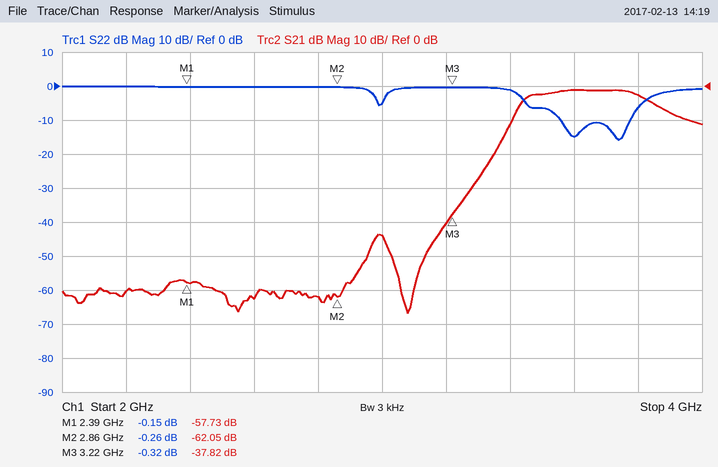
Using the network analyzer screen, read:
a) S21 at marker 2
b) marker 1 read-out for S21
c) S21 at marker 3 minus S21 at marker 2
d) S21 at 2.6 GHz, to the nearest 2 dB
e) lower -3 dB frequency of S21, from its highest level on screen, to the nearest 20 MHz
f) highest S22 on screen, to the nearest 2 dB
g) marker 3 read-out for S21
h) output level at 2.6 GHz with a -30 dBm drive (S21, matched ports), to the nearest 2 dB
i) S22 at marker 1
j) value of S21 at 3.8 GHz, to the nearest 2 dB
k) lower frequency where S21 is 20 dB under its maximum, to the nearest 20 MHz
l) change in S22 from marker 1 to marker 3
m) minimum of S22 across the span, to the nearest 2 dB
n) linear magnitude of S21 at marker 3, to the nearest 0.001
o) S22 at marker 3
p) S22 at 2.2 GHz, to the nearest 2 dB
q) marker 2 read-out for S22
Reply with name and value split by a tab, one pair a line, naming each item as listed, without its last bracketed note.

S21 at marker 2	-62.05 dB
marker 1 read-out for S21	-57.73 dB
S21 at marker 3 minus S21 at marker 2	24.23 dB
S21 at 2.6 GHz, to the nearest 2 dB	-62 dB
lower -3 dB frequency of S21, from its highest level on screen, to the nearest 20 MHz	3.44 GHz
highest S22 on screen, to the nearest 2 dB	0 dB
marker 3 read-out for S21	-37.82 dB
output level at 2.6 GHz with a -30 dBm drive (S21, matched ports), to the nearest 2 dB	-92 dBm
S22 at marker 1	-0.15 dB
value of S21 at 3.8 GHz, to the nearest 2 dB	-2 dB
lower frequency where S21 is 20 dB under its maximum, to the nearest 20 MHz	3.34 GHz
change in S22 from marker 1 to marker 3	-0.17 dB
minimum of S22 across the span, to the nearest 2 dB	-16 dB
linear magnitude of S21 at marker 3, to the nearest 0.001	0.013
S22 at marker 3	-0.32 dB
S22 at 2.2 GHz, to the nearest 2 dB	0 dB
marker 2 read-out for S22	-0.26 dB
